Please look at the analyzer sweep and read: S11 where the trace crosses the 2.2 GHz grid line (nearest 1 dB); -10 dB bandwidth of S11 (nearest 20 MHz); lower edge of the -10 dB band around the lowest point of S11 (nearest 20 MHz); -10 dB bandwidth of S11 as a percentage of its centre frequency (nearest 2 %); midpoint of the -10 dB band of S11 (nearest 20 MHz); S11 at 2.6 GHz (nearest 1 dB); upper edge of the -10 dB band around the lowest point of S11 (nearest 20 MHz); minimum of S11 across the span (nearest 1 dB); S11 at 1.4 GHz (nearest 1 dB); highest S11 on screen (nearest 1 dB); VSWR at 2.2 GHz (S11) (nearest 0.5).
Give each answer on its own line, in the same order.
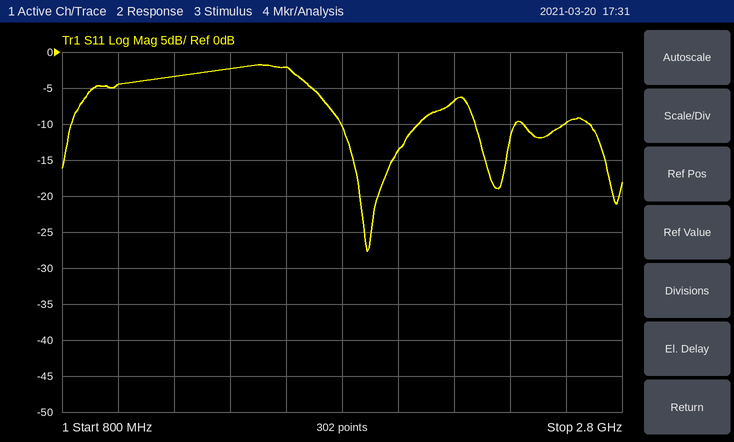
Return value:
-7 dB
280 MHz
1.80 GHz
14 %
1.94 GHz
-10 dB
2.08 GHz
-28 dB
-2 dB
-2 dB
2.5
